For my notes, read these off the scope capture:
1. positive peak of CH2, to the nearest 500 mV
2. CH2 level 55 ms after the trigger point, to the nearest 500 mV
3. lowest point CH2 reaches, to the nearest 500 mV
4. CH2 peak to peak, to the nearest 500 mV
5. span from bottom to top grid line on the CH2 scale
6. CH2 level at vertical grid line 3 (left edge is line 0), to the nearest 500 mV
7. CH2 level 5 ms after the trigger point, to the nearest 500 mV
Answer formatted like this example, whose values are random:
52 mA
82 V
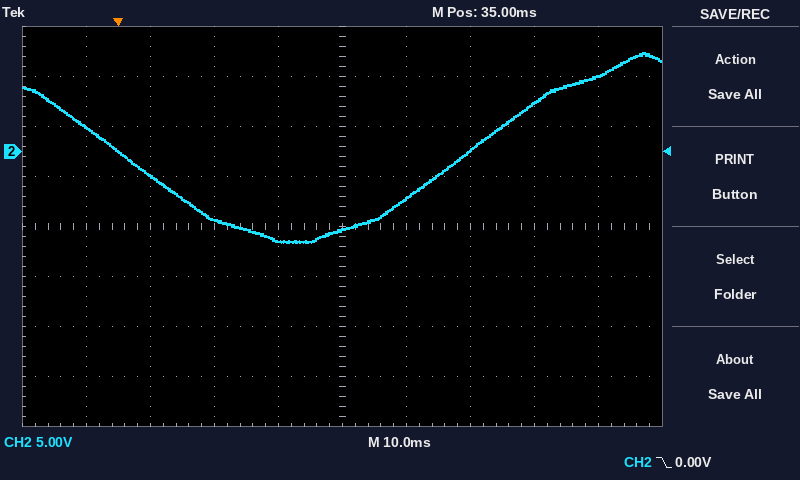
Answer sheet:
10.0 V
0.0 V
-9.0 V
19.0 V
40 V
-7.0 V
-2.5 V
